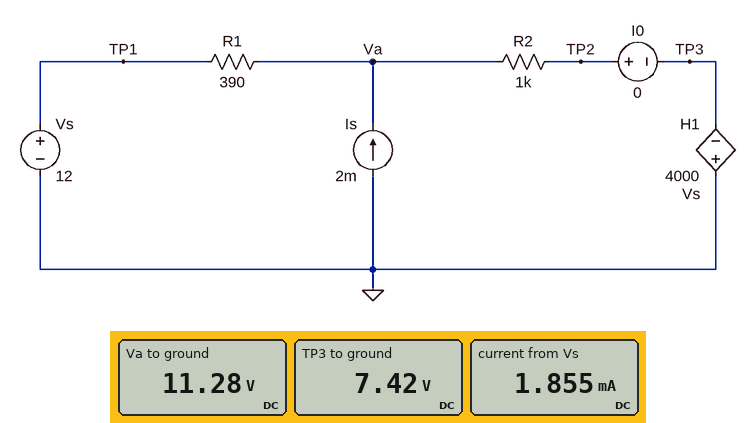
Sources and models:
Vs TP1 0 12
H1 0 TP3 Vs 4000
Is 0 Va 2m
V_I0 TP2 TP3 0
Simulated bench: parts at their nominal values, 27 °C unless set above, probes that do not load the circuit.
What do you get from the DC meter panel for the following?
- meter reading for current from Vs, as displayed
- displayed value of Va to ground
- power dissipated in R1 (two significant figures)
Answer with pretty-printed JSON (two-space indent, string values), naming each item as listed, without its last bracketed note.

{
  "meter reading for current from Vs, as displayed": "1.855 mA",
  "displayed value of Va to ground": "11.28 V",
  "power dissipated in R1": "1.3 mW"
}
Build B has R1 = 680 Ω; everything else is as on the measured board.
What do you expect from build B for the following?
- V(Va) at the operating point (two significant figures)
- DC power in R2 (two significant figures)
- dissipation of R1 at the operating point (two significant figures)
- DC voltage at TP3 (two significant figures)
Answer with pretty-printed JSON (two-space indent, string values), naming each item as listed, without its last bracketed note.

{
  "V(Va) at the operating point": "11 V",
  "DC power in R2": "14 mW",
  "dissipation of R1 at the operating point": "2.1 mW",
  "DC voltage at TP3": "7.0 V"
}
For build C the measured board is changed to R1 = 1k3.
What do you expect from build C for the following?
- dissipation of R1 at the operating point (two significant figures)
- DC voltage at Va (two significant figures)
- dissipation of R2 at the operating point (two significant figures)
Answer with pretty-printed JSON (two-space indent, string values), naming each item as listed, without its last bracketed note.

{
  "dissipation of R1 at the operating point": "3.3 mW",
  "DC voltage at Va": "9.9 V",
  "dissipation of R2 at the operating point": "13 mW"
}
